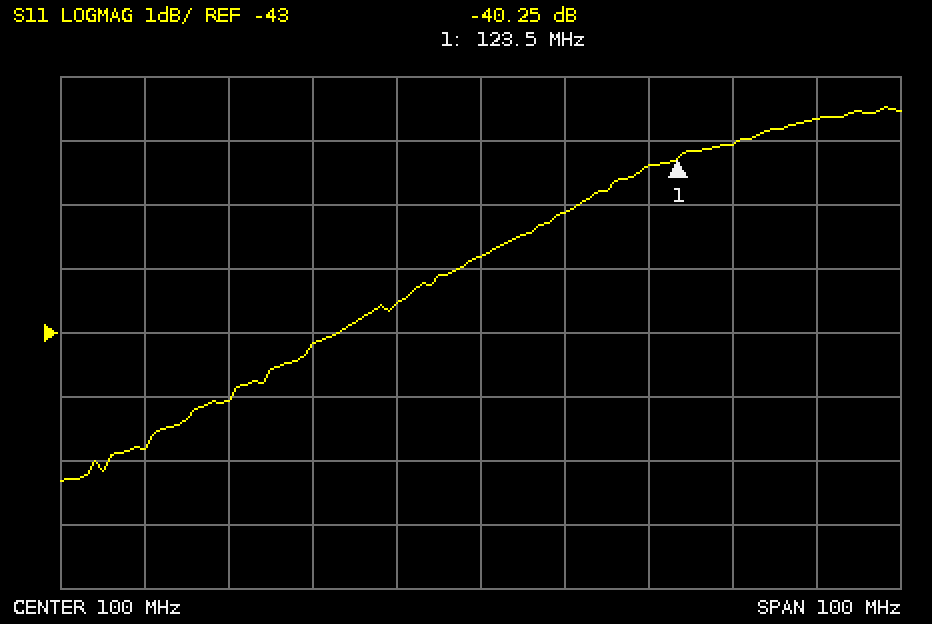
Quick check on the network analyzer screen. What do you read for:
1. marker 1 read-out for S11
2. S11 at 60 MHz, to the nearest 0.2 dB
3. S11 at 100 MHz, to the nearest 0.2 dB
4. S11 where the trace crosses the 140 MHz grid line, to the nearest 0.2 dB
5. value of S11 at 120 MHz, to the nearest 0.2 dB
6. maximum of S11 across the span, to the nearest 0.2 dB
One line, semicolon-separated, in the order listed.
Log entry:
-40.25 dB; -44.8 dB; -41.8 dB; -39.6 dB; -40.4 dB; -39.4 dB
